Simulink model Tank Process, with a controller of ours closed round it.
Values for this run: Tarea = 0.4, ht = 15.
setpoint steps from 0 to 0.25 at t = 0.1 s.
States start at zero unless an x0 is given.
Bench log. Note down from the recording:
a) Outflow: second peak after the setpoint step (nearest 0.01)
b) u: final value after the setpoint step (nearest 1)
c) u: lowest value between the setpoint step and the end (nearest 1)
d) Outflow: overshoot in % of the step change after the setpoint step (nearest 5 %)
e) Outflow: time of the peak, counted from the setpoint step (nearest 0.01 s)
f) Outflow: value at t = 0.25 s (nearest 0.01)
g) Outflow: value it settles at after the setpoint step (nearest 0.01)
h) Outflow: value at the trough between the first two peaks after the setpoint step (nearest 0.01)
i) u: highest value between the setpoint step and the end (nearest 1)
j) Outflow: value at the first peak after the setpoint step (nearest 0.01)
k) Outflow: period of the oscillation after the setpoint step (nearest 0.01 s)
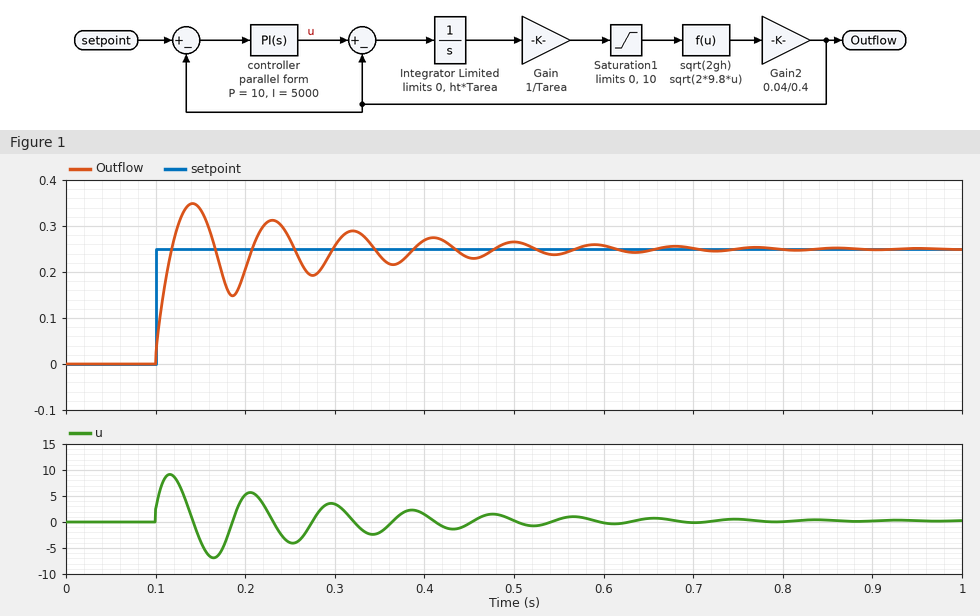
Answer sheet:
0.31
0
-7
40 %
0.04 s
0.27
0.25
0.15
9
0.35
0.09 s
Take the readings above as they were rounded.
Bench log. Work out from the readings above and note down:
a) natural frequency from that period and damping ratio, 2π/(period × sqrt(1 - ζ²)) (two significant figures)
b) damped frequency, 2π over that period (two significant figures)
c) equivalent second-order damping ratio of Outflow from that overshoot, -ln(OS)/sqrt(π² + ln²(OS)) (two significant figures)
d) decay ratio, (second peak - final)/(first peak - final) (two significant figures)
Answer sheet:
73 rad/s
70 rad/s
0.28
0.60
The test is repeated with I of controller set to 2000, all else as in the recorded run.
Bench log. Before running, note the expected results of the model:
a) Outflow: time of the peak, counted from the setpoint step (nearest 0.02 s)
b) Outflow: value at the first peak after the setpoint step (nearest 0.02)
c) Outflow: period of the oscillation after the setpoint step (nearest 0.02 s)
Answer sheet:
0.06 s
0.34
0.14 s
